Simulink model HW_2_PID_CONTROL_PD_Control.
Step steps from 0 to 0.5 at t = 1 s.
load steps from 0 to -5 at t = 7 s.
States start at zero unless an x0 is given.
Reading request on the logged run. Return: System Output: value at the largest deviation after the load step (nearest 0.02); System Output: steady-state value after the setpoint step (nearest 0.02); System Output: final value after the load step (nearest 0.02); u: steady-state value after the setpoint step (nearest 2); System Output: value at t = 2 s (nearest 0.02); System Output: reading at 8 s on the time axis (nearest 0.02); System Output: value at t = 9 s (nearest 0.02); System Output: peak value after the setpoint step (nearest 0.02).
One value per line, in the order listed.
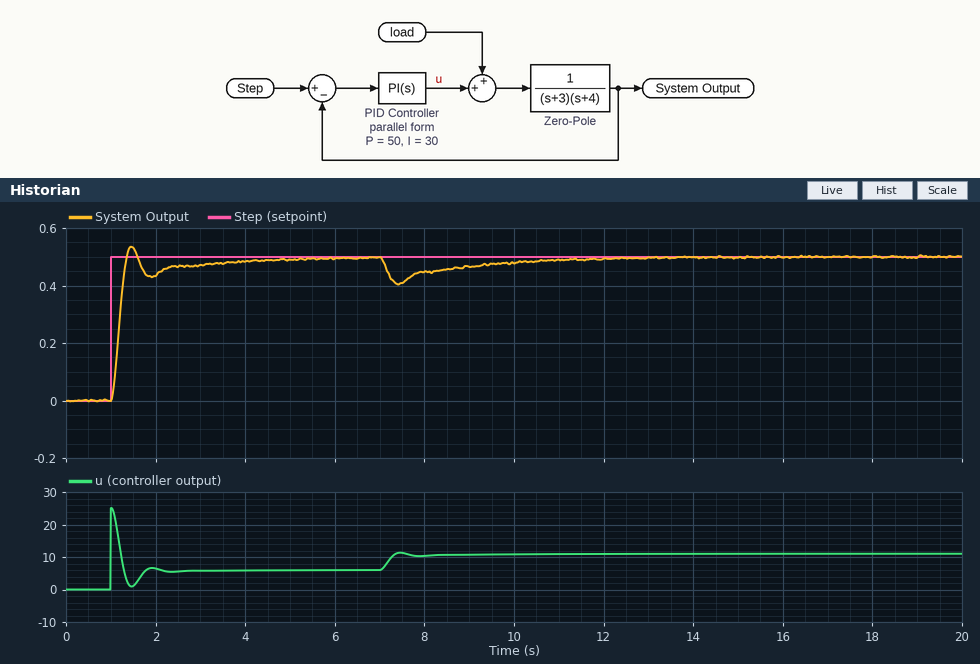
0.40
0.50
0.50
6
0.44
0.44
0.46
0.54
